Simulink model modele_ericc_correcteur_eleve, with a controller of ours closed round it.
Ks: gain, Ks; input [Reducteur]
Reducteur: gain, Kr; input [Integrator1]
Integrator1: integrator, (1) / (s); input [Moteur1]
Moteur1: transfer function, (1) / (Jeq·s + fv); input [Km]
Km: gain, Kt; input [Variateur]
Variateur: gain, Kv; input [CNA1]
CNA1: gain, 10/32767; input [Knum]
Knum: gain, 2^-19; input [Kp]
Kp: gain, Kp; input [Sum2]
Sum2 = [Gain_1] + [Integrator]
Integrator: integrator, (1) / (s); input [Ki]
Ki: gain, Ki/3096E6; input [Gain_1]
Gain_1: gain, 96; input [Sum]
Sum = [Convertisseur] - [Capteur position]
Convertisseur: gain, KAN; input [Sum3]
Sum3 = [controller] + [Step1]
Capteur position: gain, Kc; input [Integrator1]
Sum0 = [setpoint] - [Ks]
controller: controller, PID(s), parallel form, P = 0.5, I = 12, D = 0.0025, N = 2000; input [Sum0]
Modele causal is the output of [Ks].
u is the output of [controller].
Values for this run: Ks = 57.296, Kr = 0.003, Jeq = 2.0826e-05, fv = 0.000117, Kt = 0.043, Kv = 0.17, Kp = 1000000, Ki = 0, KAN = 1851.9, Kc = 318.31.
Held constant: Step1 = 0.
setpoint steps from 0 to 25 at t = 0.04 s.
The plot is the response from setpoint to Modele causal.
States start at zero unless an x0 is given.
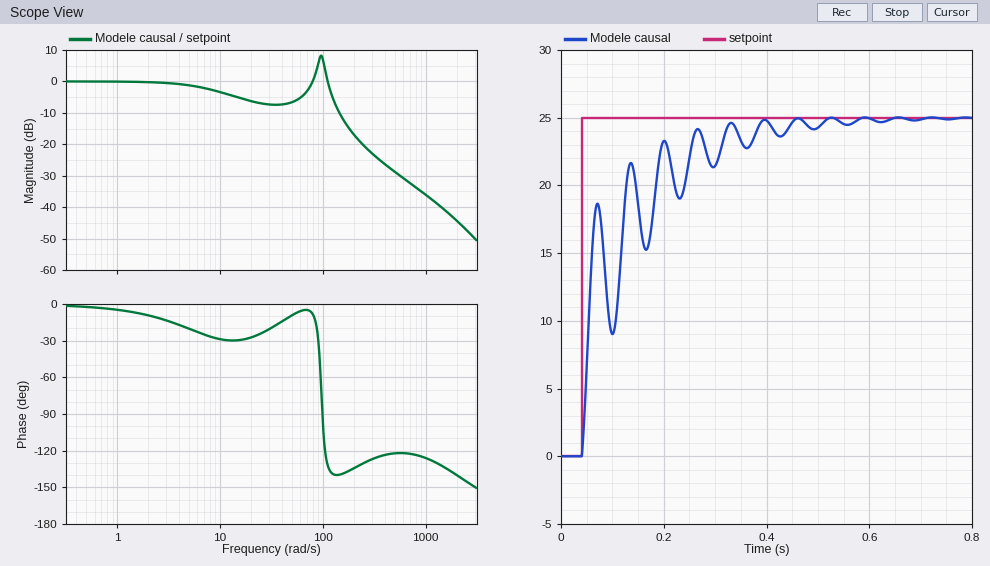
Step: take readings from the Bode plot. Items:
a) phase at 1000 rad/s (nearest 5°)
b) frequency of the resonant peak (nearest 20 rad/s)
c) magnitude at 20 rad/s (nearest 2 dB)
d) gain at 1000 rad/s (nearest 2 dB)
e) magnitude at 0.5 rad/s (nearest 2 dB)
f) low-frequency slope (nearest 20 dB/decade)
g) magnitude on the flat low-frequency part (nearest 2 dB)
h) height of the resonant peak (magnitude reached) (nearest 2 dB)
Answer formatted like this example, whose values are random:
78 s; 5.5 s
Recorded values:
-125°; 100 rad/s; -6 dB; -36 dB; 0 dB; 0 dB/decade; 0 dB; 8 dB
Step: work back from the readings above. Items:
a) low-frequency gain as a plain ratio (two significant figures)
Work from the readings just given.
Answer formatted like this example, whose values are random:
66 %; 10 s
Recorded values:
1.0
